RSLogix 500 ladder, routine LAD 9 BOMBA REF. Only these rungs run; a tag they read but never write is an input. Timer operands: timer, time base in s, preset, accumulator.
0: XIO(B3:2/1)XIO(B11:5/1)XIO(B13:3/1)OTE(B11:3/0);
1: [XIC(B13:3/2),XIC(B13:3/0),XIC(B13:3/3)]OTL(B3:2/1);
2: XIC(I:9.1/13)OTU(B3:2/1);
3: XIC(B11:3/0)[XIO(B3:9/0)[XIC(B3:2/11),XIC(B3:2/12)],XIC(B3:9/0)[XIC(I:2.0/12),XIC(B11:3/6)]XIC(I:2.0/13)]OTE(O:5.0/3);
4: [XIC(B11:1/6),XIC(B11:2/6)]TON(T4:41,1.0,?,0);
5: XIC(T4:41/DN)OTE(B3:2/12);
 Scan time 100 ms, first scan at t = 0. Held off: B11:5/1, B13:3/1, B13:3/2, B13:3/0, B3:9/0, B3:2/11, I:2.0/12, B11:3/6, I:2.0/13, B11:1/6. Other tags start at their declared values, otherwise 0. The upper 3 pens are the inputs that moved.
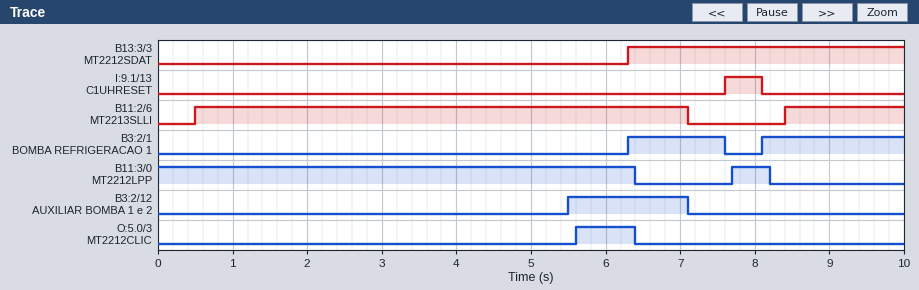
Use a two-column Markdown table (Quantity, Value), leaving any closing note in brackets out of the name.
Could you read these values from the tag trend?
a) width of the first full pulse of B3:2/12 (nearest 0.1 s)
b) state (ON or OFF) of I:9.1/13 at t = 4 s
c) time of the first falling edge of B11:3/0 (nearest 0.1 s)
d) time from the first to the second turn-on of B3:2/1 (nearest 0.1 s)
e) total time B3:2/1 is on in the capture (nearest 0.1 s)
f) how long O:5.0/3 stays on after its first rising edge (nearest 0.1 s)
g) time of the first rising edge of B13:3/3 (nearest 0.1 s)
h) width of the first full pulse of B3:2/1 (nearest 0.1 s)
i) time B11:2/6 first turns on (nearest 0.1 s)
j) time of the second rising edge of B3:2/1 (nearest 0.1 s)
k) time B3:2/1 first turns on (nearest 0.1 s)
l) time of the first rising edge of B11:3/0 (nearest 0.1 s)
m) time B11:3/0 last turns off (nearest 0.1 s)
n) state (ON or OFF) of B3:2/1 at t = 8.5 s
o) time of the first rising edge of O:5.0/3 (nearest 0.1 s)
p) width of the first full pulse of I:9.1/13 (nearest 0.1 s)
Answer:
| Quantity | Value |
|---|---|
| width of the first full pulse of B3:2/12 | 1.6 s |
| state (ON or OFF) of I:9.1/13 at t = 4 s | OFF |
| time of the first falling edge of B11:3/0 | 6.4 s |
| time from the first to the second turn-on of B3:2/1 | 1.8 s |
| total time B3:2/1 is on in the capture | 3.2 s |
| how long O:5.0/3 stays on after its first rising edge | 0.8 s |
| time of the first rising edge of B13:3/3 | 6.3 s |
| width of the first full pulse of B3:2/1 | 1.3 s |
| time B11:2/6 first turns on | 0.5 s |
| time of the second rising edge of B3:2/1 | 8.1 s |
| time B3:2/1 first turns on | 6.3 s |
| time of the first rising edge of B11:3/0 | 7.7 s |
| time B11:3/0 last turns off | 8.2 s |
| state (ON or OFF) of B3:2/1 at t = 8.5 s | ON |
| time of the first rising edge of O:5.0/3 | 5.6 s |
| width of the first full pulse of I:9.1/13 | 0.5 s |
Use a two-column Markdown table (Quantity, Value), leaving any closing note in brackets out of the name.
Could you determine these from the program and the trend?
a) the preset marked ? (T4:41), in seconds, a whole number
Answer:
| Quantity | Value |
|---|---|
| the preset marked ? (T4:41), in seconds, a whole number | 5 s |
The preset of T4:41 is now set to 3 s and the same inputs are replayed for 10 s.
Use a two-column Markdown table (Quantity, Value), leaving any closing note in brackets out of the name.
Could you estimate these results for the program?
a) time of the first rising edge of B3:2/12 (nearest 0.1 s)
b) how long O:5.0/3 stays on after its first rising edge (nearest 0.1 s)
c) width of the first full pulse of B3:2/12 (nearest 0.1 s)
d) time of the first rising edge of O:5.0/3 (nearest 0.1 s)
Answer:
| Quantity | Value |
|---|---|
| time of the first rising edge of B3:2/12 | 3.5 s |
| how long O:5.0/3 stays on after its first rising edge | 2.8 s |
| width of the first full pulse of B3:2/12 | 3.6 s |
| time of the first rising edge of O:5.0/3 | 3.6 s |
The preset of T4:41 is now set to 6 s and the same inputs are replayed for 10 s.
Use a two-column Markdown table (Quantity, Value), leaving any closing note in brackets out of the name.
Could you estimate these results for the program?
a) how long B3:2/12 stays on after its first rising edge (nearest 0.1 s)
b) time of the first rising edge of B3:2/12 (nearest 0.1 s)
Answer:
| Quantity | Value |
|---|---|
| how long B3:2/12 stays on after its first rising edge | 0.6 s |
| time of the first rising edge of B3:2/12 | 6.5 s |
